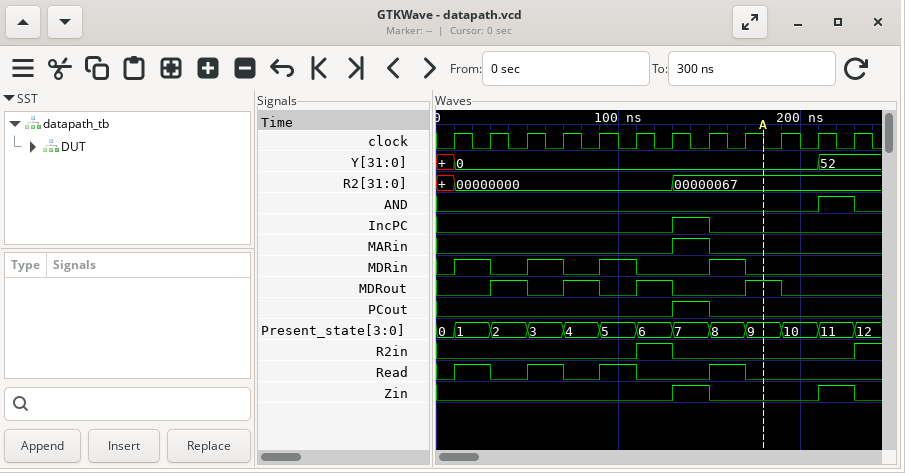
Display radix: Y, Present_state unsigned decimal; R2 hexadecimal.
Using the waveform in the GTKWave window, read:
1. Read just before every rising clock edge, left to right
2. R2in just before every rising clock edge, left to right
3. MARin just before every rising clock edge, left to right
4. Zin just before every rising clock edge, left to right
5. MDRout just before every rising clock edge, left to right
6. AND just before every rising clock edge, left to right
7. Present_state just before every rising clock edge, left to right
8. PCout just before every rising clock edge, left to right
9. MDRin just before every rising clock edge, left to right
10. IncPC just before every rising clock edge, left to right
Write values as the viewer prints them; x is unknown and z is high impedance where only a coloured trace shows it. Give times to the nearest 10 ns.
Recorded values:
0 1 0 1 0 1 0 0 1 0 0 0
0 0 0 0 0 0 1 0 0 0 0 0
0 0 0 0 0 0 0 1 0 0 0 0
0 0 0 0 0 0 0 1 0 0 0 1
0 0 1 0 1 0 1 0 0 1 0 0
0 0 0 0 0 0 0 0 0 0 0 1
0, 1, 2, 3, 4, 5, 6, 7, 8, 9, 10, 11
0 0 0 0 0 0 0 1 0 0 0 0
0 1 0 1 0 1 0 0 1 0 0 0
0 0 0 0 0 0 0 1 0 0 0 0
